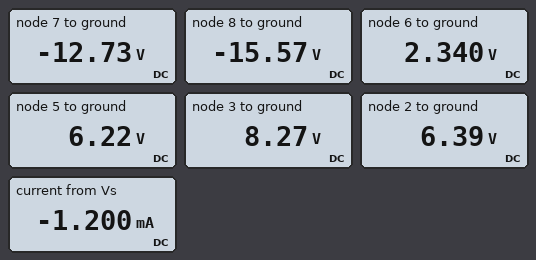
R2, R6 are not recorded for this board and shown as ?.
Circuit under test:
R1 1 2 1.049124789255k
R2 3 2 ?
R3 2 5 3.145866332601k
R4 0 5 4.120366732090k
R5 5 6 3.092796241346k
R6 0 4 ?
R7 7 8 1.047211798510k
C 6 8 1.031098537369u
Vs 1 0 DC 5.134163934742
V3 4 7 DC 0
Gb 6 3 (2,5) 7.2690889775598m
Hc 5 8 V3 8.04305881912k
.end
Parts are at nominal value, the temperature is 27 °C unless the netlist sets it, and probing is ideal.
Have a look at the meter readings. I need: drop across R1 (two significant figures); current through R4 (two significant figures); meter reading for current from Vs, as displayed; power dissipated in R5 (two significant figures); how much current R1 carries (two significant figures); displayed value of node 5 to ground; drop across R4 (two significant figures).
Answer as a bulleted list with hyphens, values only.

- 1.3 V
- 1.5 mA
- -1.200 mA
- 4.9 mW
- 1.2 mA
- 6.22 V
- 6.2 V
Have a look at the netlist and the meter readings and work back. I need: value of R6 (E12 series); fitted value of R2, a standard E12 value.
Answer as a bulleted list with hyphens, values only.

- 4.7 kΩ
- 1.5 kΩ
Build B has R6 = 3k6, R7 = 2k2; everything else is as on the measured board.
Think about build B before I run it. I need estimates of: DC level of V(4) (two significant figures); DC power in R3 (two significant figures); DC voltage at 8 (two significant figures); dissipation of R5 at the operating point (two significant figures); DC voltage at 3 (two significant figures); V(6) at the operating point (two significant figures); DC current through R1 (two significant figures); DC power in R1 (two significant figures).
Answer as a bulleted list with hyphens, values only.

- -10 V
- 11 µW
- -16 V
- 5.5 mW
- 8.5 V
- 2.2 V
- 1.3 mA
- 1.7 mW
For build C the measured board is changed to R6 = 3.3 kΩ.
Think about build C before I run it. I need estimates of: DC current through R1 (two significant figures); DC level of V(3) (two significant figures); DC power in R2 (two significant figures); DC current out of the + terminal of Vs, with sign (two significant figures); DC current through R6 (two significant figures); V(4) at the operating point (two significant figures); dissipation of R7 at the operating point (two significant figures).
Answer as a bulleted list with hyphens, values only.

- 150 µA
- 5.5 V
- 35 µW
- -150 µA
- 1.4 mA
- -4.7 V
- 2.1 mW
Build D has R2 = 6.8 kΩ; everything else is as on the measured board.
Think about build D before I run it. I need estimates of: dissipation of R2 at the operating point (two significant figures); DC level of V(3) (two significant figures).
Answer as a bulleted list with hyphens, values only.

- 11 mW
- 15 V
